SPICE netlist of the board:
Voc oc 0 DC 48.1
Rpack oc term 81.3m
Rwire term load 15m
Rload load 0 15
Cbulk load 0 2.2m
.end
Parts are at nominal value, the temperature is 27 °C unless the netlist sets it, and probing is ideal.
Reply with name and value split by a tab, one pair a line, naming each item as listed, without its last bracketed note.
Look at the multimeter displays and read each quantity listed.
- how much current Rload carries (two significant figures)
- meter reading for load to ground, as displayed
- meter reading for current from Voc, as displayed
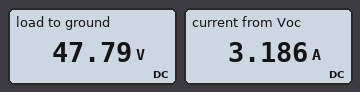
how much current Rload carries	3.2 A
meter reading for load to ground, as displayed	47.79 V
meter reading for current from Voc, as displayed	3.186 A
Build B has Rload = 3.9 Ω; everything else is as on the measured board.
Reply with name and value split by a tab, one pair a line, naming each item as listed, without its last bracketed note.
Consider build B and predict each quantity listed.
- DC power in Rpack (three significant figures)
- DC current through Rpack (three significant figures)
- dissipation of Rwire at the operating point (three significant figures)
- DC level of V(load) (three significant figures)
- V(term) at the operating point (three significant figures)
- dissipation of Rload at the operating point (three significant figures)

DC power in Rpack	11.8 W
DC current through Rpack	12.0 A
dissipation of Rwire at the operating point	2.17 W
DC level of V(load)	46.9 V
V(term) at the operating point	47.1 V
dissipation of Rload at the operating point	565 W
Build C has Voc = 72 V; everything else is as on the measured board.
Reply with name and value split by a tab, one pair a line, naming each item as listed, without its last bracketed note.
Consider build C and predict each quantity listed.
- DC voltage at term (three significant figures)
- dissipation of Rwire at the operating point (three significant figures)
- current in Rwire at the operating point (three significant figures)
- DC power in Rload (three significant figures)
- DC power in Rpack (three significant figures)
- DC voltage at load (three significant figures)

DC voltage at term	71.6 V
dissipation of Rwire at the operating point	341 mW
current in Rwire at the operating point	4.77 A
DC power in Rload	341 W
DC power in Rpack	1.85 W
DC voltage at load	71.5 V
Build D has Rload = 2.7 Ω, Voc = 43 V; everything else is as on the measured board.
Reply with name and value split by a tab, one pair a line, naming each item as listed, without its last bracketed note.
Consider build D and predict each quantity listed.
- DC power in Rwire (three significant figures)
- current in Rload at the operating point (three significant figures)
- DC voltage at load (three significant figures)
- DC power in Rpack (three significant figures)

DC power in Rwire	3.55 W
current in Rload at the operating point	15.4 A
DC voltage at load	41.5 V
DC power in Rpack	19.2 W
